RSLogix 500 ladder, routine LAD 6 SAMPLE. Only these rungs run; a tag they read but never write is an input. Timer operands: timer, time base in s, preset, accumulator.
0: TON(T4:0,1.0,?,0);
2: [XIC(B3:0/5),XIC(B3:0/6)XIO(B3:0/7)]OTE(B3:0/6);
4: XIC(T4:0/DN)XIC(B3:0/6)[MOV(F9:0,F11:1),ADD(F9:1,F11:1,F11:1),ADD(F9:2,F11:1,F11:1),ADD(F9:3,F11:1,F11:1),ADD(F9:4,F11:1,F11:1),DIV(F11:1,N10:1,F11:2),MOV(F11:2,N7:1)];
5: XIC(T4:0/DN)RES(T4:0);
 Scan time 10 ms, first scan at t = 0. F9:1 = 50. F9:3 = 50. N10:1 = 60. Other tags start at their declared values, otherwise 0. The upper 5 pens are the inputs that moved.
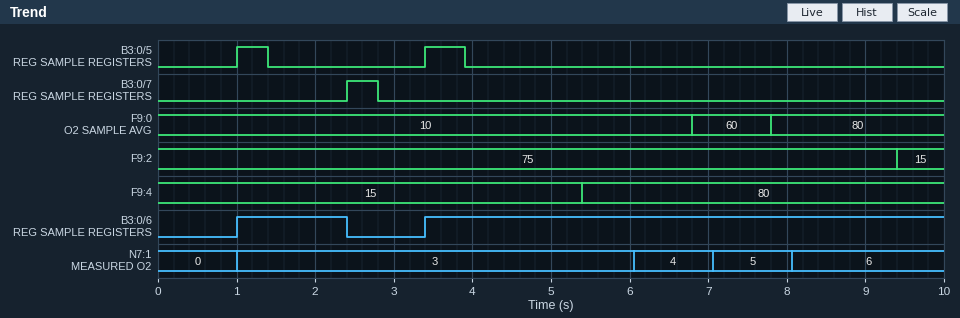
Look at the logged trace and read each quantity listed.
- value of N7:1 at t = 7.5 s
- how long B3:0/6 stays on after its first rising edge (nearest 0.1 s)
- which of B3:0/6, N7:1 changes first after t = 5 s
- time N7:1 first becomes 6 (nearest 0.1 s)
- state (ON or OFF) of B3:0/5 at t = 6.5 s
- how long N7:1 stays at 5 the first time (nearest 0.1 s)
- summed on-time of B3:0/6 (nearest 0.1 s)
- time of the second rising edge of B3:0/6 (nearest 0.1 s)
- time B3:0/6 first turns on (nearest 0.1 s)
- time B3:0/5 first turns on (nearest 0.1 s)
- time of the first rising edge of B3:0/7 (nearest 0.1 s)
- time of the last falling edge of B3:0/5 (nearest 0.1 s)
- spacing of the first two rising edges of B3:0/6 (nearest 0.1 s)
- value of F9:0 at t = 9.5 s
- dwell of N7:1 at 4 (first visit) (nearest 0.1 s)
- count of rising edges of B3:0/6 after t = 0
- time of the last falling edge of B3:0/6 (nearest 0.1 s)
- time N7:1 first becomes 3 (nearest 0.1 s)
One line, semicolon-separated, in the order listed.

5; 1.4 s; N7:1; 8.1 s; OFF; 1.0 s; 8.0 s; 3.4 s; 1.0 s; 1.0 s; 2.4 s; 3.9 s; 2.4 s; 80; 1.0 s; 2; 2.4 s; 1.0 s
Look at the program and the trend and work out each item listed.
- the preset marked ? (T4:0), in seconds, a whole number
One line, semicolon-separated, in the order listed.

1 s
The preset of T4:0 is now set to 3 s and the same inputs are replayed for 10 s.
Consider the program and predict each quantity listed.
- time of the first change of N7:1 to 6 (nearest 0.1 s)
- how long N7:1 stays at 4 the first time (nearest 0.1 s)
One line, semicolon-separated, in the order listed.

9.0 s; 3.0 s
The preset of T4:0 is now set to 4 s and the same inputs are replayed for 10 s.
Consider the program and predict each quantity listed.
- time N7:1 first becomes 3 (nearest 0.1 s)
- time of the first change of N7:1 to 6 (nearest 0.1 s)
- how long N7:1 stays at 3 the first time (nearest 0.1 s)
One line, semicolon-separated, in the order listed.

4.0 s; 8.0 s; 4.0 s
